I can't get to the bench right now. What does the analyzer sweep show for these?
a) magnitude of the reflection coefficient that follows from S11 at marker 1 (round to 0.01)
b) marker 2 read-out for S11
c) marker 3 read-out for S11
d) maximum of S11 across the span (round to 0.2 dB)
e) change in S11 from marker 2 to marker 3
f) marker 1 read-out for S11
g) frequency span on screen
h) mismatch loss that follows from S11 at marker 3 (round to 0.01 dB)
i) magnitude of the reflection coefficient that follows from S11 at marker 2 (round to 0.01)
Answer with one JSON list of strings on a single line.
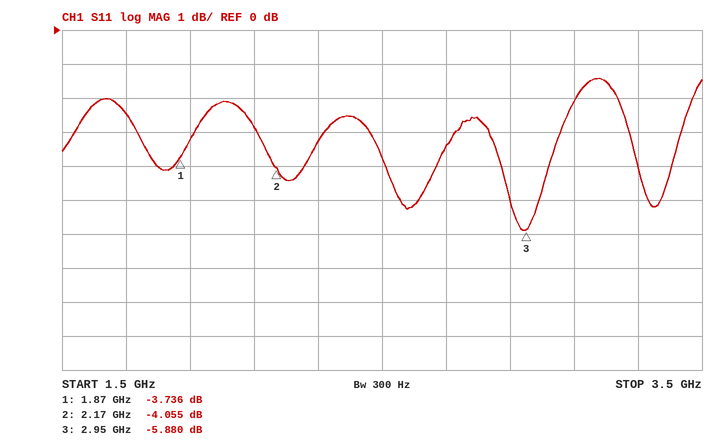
["0.65", "-4.055 dB", "-5.880 dB", "-1.4 dB", "-1.825 dB", "-3.736 dB", "2 GHz", "1.30 dB", "0.63"]
